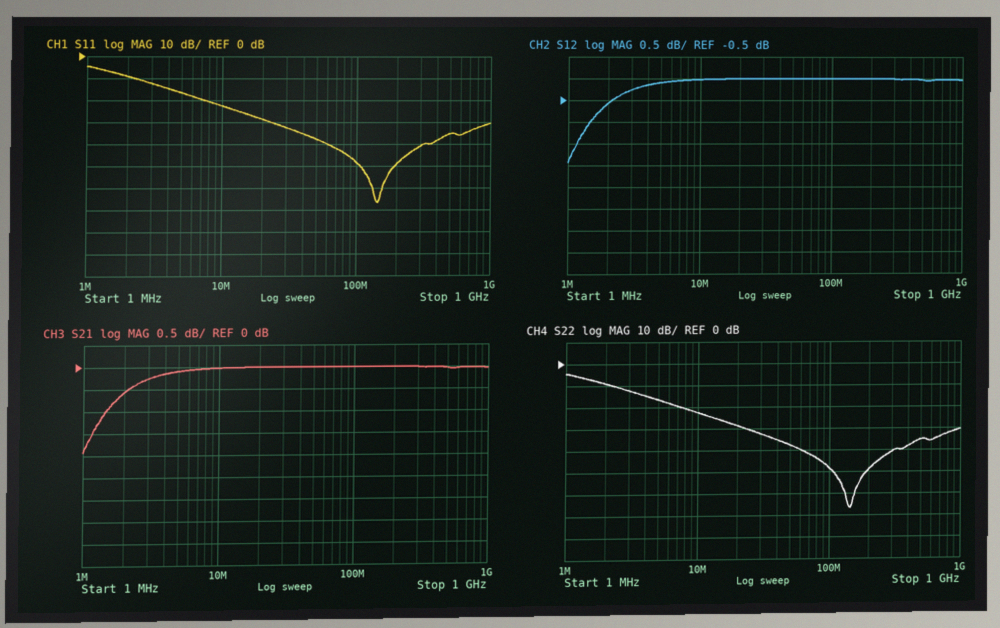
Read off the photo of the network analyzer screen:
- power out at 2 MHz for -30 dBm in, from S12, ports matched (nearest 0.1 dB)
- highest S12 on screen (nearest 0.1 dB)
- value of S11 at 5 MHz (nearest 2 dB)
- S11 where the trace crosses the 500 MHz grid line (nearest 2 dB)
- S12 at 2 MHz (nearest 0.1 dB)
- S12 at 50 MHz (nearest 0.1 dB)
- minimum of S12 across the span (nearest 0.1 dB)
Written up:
-30.6 dBm
0.0 dB
-16 dB
-36 dB
-0.6 dB
0.0 dB
-1.9 dB
